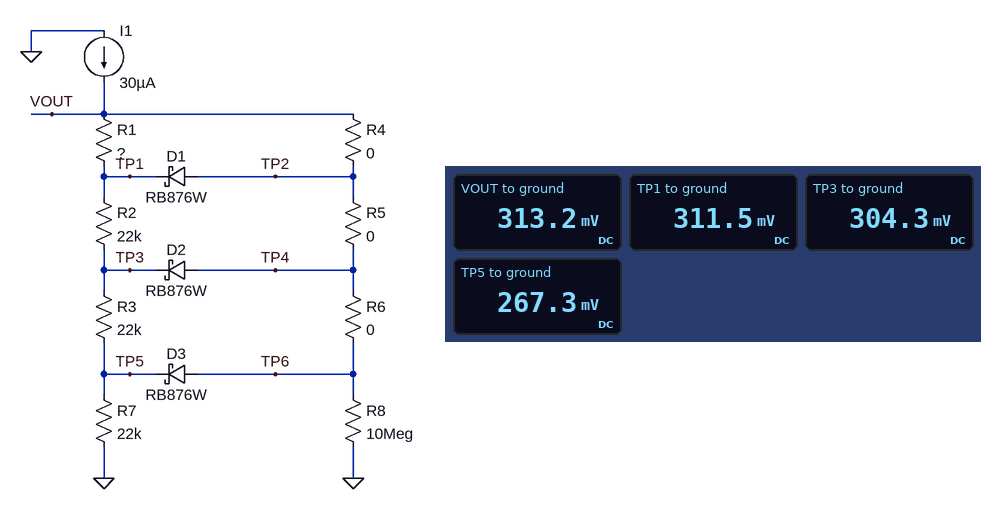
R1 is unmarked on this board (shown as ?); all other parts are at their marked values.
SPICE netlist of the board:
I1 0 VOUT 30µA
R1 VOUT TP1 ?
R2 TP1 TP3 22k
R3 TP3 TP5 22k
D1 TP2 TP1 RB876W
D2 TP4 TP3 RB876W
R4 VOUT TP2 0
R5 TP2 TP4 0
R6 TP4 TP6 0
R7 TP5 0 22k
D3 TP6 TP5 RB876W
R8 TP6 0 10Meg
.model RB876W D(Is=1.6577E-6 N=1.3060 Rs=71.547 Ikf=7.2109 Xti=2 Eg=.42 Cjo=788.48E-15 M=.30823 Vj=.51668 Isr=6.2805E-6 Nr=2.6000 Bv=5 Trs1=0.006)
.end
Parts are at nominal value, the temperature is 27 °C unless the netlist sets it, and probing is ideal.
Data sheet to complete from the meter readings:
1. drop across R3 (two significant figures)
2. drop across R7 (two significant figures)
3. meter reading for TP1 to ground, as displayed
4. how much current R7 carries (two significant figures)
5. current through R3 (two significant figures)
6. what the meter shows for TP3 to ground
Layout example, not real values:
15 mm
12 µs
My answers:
37 mV
270 mV
311.5 mV
12 µA
1.7 µA
304.3 mV
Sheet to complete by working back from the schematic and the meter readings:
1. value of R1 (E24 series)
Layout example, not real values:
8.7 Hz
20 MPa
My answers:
20 kΩ
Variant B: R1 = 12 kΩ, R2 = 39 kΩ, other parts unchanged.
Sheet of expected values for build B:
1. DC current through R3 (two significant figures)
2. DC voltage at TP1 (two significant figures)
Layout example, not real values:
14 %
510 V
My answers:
2.0 µA
390 mV
